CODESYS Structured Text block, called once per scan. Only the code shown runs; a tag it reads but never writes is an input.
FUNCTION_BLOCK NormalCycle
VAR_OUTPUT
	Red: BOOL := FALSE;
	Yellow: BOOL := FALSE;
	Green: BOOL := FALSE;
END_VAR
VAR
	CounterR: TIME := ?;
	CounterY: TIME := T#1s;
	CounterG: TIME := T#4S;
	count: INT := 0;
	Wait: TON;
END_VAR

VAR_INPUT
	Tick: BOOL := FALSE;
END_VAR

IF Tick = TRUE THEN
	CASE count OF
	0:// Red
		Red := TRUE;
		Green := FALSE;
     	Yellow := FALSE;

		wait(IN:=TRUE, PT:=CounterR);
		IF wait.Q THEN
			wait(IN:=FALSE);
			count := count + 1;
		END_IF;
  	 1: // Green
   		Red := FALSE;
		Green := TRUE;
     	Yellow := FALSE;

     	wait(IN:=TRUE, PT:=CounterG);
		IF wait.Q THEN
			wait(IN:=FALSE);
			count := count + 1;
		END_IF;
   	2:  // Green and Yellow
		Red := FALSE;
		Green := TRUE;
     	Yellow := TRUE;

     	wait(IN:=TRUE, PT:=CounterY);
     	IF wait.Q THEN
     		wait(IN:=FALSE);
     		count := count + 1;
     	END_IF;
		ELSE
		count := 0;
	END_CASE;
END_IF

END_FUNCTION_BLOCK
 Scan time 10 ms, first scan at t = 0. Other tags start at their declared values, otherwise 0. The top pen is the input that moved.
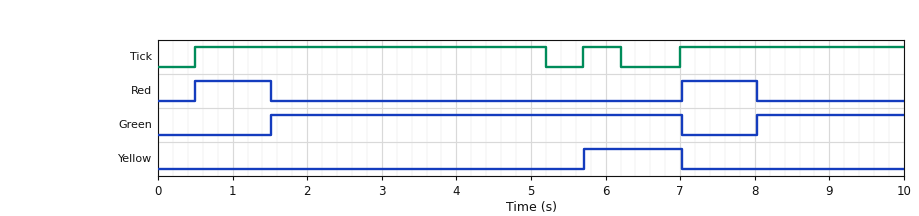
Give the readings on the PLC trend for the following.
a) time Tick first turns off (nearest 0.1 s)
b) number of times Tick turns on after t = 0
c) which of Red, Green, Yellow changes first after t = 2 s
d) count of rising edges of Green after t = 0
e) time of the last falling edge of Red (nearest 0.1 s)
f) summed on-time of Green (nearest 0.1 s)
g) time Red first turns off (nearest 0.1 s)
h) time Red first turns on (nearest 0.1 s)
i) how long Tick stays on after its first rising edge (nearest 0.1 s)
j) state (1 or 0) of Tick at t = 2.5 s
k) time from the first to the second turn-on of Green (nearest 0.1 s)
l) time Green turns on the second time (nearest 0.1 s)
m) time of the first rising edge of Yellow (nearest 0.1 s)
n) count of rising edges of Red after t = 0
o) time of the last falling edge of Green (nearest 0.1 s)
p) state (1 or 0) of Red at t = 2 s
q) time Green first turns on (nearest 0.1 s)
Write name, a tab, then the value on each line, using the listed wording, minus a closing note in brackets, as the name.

time Tick first turns off	5.2 s
number of times Tick turns on after t = 0	3
which of Red, Green, Yellow changes first after t = 2 s	Yellow
count of rising edges of Green after t = 0	2
time of the last falling edge of Red	8.0 s
summed on-time of Green	7.5 s
time Red first turns off	1.5 s
time Red first turns on	0.5 s
how long Tick stays on after its first rising edge	4.7 s
state (1 or 0) of Tick at t = 2.5 s	1
time from the first to the second turn-on of Green	6.5 s
time Green turns on the second time	8.0 s
time of the first rising edge of Yellow	5.7 s
count of rising edges of Red after t = 0	2
time of the last falling edge of Green	7.0 s
state (1 or 0) of Red at t = 2 s	0
time Green first turns on	1.5 s
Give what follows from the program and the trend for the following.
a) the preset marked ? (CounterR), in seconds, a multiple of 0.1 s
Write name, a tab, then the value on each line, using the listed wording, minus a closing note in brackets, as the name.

the preset marked ? (CounterR), in seconds, a multiple of 0.1 s	1.0 s
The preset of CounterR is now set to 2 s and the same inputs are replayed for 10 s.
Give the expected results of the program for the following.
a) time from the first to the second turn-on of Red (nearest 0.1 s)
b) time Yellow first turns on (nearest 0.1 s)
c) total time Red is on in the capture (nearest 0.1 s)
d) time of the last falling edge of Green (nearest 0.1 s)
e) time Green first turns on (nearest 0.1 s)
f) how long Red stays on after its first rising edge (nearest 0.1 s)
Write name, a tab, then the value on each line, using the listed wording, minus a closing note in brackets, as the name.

time from the first to the second turn-on of Red	7.5 s
time Yellow first turns on	7.0 s
total time Red is on in the capture	4.0 s
time of the last falling edge of Green	8.0 s
time Green first turns on	2.5 s
how long Red stays on after its first rising edge	2.0 s
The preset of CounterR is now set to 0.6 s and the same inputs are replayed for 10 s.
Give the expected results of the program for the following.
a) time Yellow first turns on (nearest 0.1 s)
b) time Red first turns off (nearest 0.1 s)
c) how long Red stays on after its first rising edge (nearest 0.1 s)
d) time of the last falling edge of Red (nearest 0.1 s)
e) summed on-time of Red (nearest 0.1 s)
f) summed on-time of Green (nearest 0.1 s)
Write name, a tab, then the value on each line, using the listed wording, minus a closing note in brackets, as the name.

time Yellow first turns on	5.1 s
time Red first turns off	1.1 s
how long Red stays on after its first rising edge	0.6 s
time of the last falling edge of Red	7.0 s
summed on-time of Red	1.5 s
summed on-time of Green	8.0 s
